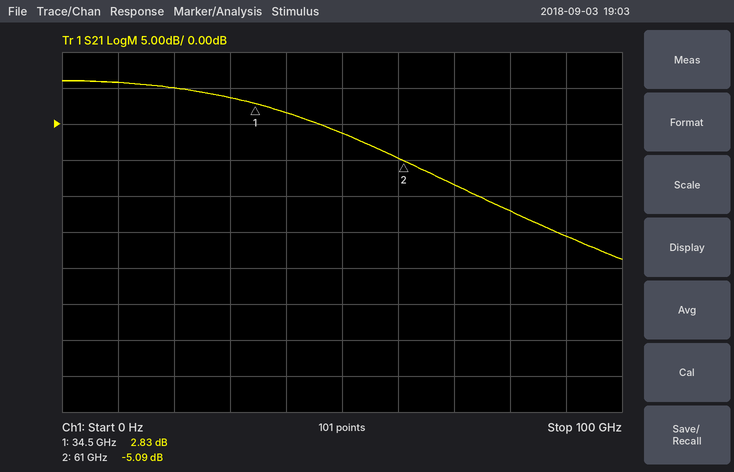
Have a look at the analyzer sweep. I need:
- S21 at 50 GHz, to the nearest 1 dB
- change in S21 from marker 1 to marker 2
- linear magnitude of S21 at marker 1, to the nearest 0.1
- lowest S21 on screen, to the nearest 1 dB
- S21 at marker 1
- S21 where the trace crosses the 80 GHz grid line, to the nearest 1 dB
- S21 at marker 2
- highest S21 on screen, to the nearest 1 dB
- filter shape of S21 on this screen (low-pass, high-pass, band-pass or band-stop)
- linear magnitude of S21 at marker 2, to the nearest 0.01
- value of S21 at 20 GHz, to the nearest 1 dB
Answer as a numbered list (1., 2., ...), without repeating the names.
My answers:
1. -1 dB
2. -7.92 dB
3. 1.4
4. -19 dB
5. 2.83 dB
6. -12 dB
7. -5.09 dB
8. 6 dB
9. low-pass
10. 0.56
11. 5 dB
